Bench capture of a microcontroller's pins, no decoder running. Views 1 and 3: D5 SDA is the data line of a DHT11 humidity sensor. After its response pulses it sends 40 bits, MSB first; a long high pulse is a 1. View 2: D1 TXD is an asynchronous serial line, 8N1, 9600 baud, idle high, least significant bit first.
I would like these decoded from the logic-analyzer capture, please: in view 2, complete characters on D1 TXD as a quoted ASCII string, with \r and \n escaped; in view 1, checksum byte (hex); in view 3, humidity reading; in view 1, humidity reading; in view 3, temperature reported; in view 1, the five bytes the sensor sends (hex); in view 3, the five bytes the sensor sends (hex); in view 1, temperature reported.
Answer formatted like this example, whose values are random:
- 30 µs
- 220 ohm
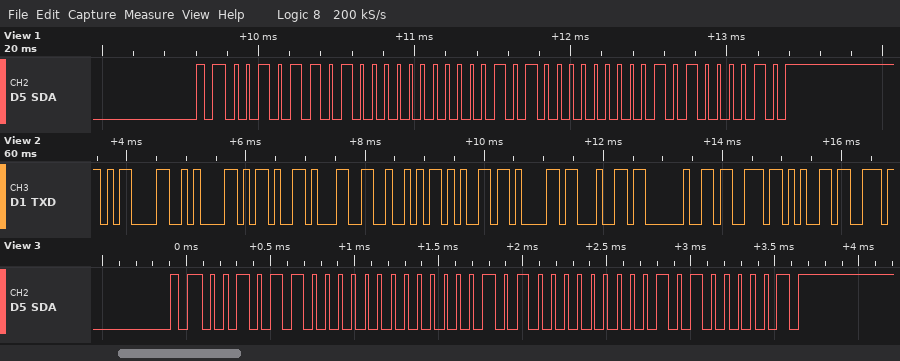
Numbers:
- "\r\n-1Read se"
- 0x42
- 44 %
- 45 %
- 20.1 °C
- 2D 00 14 01 42
- 2C 00 14 01 41
- 20.1 °C
